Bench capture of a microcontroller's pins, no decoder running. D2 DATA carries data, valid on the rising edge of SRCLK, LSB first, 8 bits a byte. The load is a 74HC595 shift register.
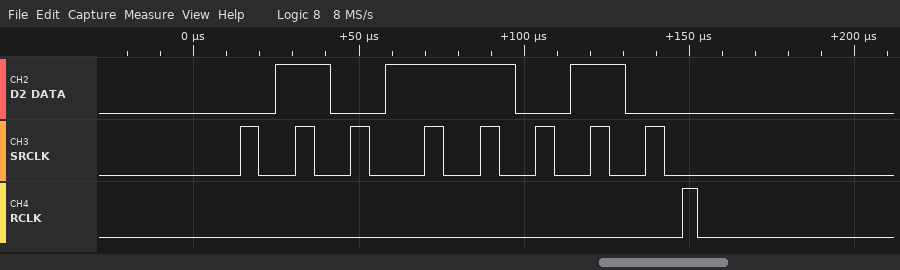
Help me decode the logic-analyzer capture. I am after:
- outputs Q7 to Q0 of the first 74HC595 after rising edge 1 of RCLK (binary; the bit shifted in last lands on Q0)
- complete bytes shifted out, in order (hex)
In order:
01011010
5A
